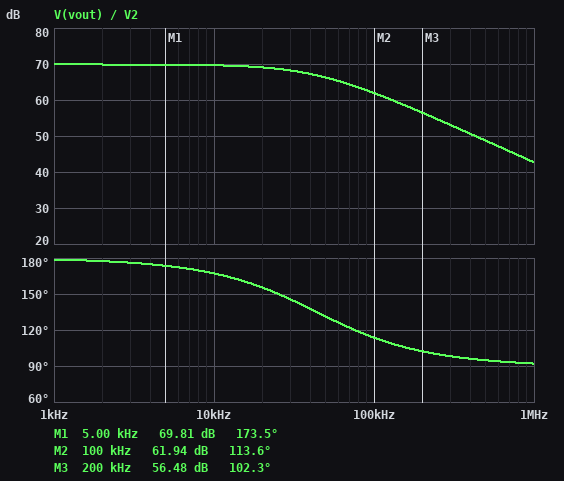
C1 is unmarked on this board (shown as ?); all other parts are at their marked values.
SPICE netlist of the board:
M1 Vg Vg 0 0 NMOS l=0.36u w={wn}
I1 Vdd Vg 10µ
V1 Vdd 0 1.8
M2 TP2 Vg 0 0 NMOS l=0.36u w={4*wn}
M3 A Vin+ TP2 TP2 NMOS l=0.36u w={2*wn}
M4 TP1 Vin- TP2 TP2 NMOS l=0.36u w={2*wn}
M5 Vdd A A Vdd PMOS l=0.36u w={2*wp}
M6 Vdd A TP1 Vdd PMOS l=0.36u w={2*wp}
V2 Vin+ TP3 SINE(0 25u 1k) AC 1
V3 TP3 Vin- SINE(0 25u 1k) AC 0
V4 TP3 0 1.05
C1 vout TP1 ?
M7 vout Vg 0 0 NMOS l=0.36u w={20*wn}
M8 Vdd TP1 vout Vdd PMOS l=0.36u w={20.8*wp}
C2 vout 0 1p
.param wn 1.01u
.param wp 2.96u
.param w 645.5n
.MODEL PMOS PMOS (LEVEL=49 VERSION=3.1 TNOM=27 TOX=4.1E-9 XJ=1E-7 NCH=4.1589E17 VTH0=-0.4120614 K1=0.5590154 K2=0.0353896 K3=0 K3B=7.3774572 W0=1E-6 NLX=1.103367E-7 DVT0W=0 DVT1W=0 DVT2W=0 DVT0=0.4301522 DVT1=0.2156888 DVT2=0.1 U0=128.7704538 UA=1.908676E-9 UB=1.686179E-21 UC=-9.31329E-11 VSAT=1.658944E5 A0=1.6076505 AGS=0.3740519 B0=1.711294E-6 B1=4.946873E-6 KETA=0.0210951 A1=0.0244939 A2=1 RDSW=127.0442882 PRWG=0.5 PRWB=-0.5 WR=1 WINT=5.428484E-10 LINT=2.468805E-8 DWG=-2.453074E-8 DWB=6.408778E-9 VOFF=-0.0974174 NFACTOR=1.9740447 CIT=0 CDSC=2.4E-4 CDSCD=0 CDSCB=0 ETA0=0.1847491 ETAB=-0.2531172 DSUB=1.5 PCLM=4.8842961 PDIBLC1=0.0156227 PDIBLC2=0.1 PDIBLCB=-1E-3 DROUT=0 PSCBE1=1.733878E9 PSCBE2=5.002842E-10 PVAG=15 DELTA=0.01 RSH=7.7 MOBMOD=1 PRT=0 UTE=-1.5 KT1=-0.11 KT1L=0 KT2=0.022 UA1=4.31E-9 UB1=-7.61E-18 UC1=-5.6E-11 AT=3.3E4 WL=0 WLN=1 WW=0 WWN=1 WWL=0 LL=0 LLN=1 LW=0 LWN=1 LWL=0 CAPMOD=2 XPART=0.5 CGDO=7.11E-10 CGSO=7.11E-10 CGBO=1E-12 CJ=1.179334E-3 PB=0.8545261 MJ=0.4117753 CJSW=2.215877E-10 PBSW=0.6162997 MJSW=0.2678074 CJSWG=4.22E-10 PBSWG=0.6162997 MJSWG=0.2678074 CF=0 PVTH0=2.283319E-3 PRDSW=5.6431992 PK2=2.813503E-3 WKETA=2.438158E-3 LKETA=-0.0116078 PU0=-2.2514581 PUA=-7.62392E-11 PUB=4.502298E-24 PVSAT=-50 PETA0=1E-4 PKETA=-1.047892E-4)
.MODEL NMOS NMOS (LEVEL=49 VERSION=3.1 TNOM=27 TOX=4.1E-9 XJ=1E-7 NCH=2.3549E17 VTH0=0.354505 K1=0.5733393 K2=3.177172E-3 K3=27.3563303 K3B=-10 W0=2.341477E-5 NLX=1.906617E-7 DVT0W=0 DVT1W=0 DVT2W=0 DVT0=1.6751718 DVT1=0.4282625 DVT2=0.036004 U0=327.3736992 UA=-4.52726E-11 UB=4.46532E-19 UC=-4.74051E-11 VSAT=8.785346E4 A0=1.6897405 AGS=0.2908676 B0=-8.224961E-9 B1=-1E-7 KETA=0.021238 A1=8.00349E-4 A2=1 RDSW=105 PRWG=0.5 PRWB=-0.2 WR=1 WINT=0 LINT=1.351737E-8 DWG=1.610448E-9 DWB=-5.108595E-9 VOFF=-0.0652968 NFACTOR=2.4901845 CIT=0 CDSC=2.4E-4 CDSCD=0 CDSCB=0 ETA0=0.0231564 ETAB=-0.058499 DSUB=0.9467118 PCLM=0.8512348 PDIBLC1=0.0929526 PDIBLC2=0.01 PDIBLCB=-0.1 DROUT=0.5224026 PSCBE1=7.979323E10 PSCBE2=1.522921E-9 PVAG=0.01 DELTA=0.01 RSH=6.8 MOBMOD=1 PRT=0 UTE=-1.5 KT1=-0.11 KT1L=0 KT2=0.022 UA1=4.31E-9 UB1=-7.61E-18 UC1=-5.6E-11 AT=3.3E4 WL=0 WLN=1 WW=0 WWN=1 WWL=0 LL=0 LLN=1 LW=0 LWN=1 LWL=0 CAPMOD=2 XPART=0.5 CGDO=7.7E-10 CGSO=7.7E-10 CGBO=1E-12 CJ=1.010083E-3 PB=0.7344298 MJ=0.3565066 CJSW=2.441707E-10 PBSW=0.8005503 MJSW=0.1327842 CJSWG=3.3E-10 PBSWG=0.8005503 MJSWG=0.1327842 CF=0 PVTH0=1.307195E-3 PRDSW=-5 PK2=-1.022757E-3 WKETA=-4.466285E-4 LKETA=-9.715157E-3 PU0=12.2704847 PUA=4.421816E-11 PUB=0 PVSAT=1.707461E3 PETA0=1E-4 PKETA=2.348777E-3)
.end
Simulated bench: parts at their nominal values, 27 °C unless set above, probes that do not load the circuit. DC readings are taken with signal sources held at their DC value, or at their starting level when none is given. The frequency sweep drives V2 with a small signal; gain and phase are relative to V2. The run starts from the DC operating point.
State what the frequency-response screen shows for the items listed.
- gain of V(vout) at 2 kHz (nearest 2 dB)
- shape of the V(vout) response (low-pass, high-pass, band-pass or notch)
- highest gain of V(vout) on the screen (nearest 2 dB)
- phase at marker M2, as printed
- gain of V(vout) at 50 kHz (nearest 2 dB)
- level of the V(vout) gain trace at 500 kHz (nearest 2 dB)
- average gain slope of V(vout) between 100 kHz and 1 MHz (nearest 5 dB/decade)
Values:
70 dB
low-pass
70 dB
113.6 deg
66 dB
48 dB
-20 dB/decade
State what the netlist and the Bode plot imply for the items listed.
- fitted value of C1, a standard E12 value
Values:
220 fF
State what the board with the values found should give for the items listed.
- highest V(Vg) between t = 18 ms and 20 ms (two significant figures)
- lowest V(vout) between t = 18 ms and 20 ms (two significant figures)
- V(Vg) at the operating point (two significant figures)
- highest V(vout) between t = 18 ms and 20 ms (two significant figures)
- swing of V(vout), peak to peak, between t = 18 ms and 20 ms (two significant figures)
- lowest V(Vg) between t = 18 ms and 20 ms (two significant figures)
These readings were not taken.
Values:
650 mV
760 mV
650 mV
1.1 V
310 mV
650 mV
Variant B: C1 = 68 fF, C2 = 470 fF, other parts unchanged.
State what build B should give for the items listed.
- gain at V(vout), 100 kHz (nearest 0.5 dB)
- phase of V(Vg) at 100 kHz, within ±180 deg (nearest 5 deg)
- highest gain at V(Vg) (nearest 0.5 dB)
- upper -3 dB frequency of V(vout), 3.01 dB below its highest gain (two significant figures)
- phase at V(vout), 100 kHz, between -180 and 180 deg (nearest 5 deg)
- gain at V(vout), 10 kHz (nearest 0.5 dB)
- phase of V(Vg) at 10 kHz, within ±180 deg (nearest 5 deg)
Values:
67.0 dB
-135 deg
-12.0 dB
100 kHz
135 deg
70.0 dB
-95 deg
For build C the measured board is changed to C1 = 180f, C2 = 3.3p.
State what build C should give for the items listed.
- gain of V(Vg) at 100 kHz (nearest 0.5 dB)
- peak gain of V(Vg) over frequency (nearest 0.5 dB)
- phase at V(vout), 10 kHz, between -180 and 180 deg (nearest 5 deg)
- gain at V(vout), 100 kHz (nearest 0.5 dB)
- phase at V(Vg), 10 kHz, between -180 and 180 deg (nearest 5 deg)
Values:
-19.0 dB
-18.0 dB
170 deg
63.0 dB
-100 deg
